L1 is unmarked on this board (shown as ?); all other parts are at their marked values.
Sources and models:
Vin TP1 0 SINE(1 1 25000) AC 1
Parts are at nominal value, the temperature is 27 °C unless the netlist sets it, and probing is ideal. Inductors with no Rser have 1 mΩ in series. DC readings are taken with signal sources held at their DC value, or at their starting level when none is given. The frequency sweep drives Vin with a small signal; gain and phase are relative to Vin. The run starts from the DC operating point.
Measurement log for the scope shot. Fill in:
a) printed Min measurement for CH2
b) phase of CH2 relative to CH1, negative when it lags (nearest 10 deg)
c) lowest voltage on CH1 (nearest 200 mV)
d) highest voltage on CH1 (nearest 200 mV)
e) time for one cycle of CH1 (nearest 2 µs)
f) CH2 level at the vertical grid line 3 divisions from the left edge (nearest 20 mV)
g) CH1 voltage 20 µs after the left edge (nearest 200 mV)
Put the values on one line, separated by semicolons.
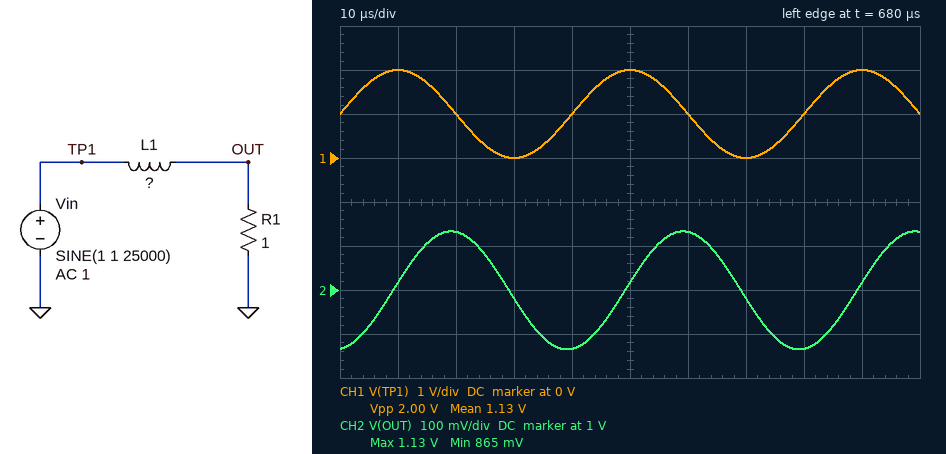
865 mV; -80 deg; 0 V; 2.0 V; 40 µs; 980 mV; 1.0 V
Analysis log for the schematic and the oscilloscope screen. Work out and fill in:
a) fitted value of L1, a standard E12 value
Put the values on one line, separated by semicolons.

47 µH
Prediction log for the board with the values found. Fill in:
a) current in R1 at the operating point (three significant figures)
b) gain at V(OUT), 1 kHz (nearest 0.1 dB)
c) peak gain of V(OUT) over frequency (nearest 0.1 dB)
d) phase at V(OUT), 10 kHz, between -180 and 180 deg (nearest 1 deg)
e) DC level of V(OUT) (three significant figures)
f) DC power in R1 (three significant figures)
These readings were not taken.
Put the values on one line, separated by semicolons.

999 mA; -0.4 dB; 0 dB; -71 deg; 999 mV; 998 mW
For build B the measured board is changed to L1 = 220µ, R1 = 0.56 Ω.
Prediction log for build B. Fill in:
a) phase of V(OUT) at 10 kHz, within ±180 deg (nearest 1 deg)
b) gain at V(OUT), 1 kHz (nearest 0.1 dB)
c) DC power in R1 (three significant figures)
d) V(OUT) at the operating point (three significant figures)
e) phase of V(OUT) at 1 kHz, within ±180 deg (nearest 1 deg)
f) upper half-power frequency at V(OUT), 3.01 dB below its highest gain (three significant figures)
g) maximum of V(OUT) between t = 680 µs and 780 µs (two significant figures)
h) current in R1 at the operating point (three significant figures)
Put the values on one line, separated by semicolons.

-88 deg; -8.5 dB; 1.78 W; 998 mV; -68 deg; 406 Hz; 1.0 V; 1.78 A
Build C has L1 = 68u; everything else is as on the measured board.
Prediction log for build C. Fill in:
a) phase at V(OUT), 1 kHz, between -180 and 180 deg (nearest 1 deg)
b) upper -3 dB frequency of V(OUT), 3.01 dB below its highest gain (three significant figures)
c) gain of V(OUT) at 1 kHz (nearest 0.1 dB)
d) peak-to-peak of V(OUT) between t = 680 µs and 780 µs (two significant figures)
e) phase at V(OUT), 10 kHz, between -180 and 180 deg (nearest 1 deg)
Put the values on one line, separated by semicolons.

-23 deg; 2.34 kHz; -0.7 dB; 190 mV; -77 deg
